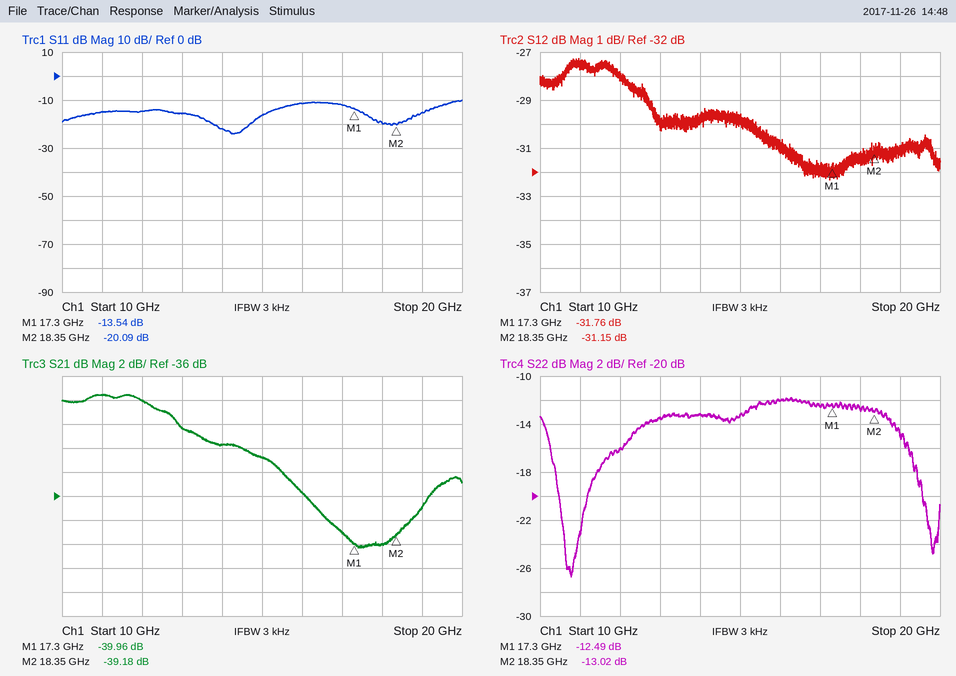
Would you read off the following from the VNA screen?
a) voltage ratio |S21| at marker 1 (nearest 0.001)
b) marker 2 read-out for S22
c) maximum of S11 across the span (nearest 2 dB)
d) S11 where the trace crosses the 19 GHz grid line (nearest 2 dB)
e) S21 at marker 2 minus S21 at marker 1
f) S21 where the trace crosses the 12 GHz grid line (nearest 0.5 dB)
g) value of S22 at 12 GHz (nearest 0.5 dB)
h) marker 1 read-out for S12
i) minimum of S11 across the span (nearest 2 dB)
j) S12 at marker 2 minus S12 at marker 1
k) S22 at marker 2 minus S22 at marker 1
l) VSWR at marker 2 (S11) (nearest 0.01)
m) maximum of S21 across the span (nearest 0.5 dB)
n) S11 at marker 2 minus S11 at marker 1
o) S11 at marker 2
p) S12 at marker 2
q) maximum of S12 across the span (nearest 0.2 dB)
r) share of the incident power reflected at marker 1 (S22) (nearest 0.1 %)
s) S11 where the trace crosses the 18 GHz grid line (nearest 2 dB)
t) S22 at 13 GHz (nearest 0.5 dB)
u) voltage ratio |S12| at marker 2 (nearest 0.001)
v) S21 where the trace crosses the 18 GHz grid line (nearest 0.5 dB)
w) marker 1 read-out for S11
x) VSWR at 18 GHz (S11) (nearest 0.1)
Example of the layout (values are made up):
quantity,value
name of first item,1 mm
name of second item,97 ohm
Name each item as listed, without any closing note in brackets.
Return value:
quantity,value
voltage ratio |S21| at marker 1,0.010
marker 2 read-out for S22,-13.02 dB
maximum of S11 across the span,-10 dB
S11 where the trace crosses the 19 GHz grid line,-16 dB
S21 at marker 2 minus S21 at marker 1,0.78 dB
S21 where the trace crosses the 12 GHz grid line,-28.0 dB
value of S22 at 12 GHz,-16.0 dB
marker 1 read-out for S12,-31.76 dB
minimum of S11 across the span,-24 dB
S12 at marker 2 minus S12 at marker 1,0.61 dB
S22 at marker 2 minus S22 at marker 1,-0.53 dB
VSWR at marker 2 (S11),1.22
maximum of S21 across the span,-27.5 dB
S11 at marker 2 minus S11 at marker 1,-6.55 dB
S11 at marker 2,-20.09 dB
S12 at marker 2,-31.15 dB
maximum of S12 across the span,-27.2 dB
share of the incident power reflected at marker 1 (S22),5.6 %
S11 where the trace crosses the 18 GHz grid line,-20 dB
S22 at 13 GHz,-13.5 dB
voltage ratio |S12| at marker 2,0.028
S21 where the trace crosses the 18 GHz grid line,-40.0 dB
marker 1 read-out for S11,-13.54 dB
VSWR at 18 GHz (S11),1.2
